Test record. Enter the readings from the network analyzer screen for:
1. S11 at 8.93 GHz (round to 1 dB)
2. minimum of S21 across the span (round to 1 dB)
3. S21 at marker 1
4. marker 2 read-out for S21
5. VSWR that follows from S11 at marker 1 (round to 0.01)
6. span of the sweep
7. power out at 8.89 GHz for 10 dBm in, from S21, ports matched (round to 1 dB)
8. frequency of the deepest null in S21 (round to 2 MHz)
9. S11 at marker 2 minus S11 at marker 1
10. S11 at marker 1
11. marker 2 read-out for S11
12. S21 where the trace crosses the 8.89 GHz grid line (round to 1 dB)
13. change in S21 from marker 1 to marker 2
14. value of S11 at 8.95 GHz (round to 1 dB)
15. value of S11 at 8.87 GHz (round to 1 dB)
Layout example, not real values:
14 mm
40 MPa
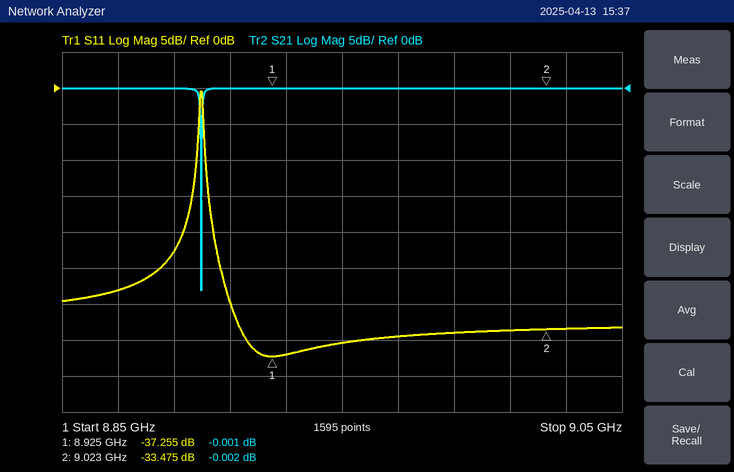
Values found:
-37 dB
-28 dB
-0.001 dB
-0.002 dB
1.03
200 MHz
10 dBm
8.900 GHz
3.780 dB
-37.255 dB
-33.475 dB
0 dB
-0.001 dB
-35 dB
-28 dB
